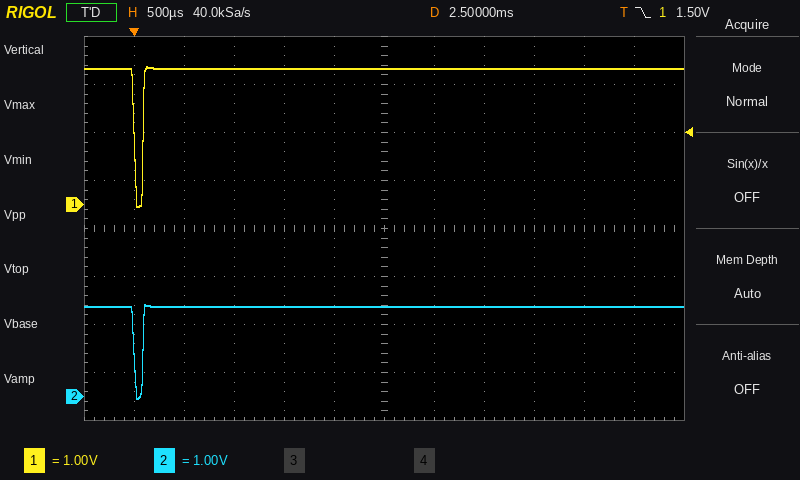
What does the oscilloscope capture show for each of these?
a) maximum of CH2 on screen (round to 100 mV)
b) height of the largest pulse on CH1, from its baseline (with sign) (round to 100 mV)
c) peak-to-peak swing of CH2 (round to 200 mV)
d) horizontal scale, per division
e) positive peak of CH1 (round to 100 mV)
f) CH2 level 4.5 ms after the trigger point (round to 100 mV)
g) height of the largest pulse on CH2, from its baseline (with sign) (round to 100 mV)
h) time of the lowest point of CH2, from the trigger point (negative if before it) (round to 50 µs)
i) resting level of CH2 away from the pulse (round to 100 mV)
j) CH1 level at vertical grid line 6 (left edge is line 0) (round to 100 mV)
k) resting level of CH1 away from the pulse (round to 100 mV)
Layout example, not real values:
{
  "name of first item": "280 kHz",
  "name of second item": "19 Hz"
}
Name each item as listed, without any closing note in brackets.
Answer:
{
  "maximum of CH2 on screen": "1.9 V",
  "height of the largest pulse on CH1, from its baseline (with sign)": "-2.9 V",
  "peak-to-peak swing of CH2": "2.0 V",
  "horizontal scale, per division": "500 µs",
  "positive peak of CH1": "2.9 V",
  "CH2 level 4.5 ms after the trigger point": "1.9 V",
  "height of the largest pulse on CH2, from its baseline (with sign)": "-1.9 V",
  "time of the lowest point of CH2, from the trigger point (negative if before it)": "+50 µs",
  "resting level of CH2 away from the pulse": "1.9 V",
  "CH1 level at vertical grid line 6 (left edge is line 0)": "2.8 V",
  "resting level of CH1 away from the pulse": "2.8 V"
}
